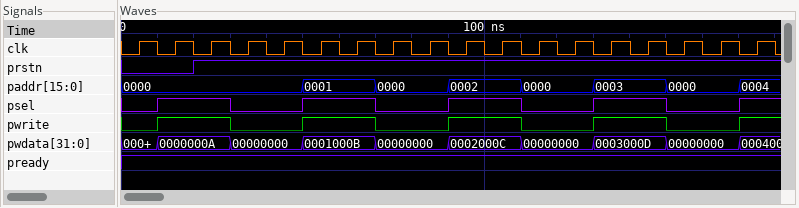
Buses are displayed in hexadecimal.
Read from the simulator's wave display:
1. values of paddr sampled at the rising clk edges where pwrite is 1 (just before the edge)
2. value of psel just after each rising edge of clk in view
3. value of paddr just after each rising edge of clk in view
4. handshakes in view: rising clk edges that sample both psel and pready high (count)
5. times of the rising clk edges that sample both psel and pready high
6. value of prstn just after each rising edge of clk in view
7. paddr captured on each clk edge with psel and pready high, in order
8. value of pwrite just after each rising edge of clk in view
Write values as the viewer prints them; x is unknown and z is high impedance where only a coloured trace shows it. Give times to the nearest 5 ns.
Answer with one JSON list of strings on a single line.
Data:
["0000, 0000, 0001, 0001, 0002, 0002, 0003, 0003, 0004", "0 1 1 0 0 1 1 0 0 1 1 0 0 1 1 0 0 1", "0000, 0000, 0000, 0000, 0000, 0001, 0001, 0000, 0000, 0002, 0002, 0000, 0000, 0003, 0003, 0000, 0000, 0004", "9", "15 ns, 25 ns, 55 ns, 65 ns, 95 ns, 105 ns, 135 ns, 145 ns, 175 ns", "0 0 1 1 1 1 1 1 1 1 1 1 1 1 1 1 1 1", "0000, 0000, 0001, 0001, 0002, 0002, 0003, 0003, 0004", "0 1 1 0 0 1 1 0 0 1 1 0 0 1 1 0 0 1"]
